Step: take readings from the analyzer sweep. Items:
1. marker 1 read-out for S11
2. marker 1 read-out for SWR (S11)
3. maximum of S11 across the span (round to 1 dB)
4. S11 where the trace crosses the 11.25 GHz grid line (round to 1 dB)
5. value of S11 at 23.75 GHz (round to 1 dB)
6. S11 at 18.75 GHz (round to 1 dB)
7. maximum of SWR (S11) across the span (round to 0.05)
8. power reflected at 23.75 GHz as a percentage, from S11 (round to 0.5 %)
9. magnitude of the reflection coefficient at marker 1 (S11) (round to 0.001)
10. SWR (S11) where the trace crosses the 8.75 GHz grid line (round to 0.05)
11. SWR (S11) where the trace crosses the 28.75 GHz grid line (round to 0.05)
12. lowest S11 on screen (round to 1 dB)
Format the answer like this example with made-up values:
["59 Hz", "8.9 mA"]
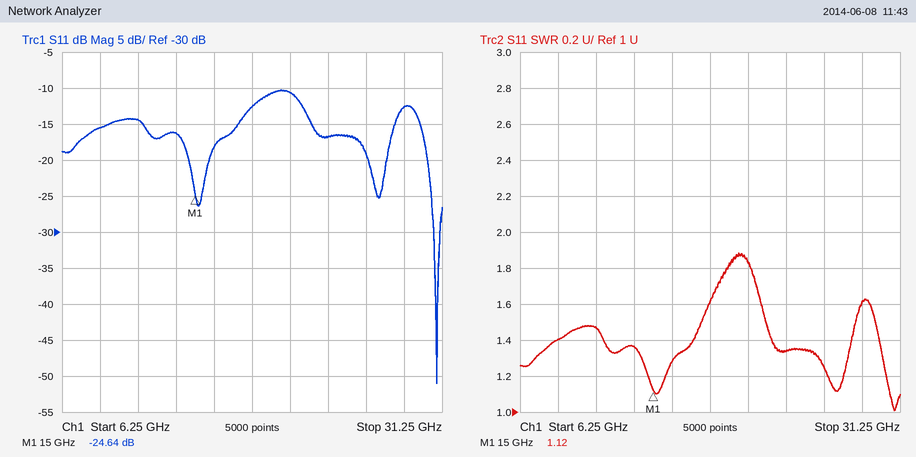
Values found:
["-24.64 dB", "1.12", "-10 dB", "-14 dB", "-17 dB", "-13 dB", "1.90", "2.0 %", "0.059", "1.40", "1.60", "-51 dB"]
